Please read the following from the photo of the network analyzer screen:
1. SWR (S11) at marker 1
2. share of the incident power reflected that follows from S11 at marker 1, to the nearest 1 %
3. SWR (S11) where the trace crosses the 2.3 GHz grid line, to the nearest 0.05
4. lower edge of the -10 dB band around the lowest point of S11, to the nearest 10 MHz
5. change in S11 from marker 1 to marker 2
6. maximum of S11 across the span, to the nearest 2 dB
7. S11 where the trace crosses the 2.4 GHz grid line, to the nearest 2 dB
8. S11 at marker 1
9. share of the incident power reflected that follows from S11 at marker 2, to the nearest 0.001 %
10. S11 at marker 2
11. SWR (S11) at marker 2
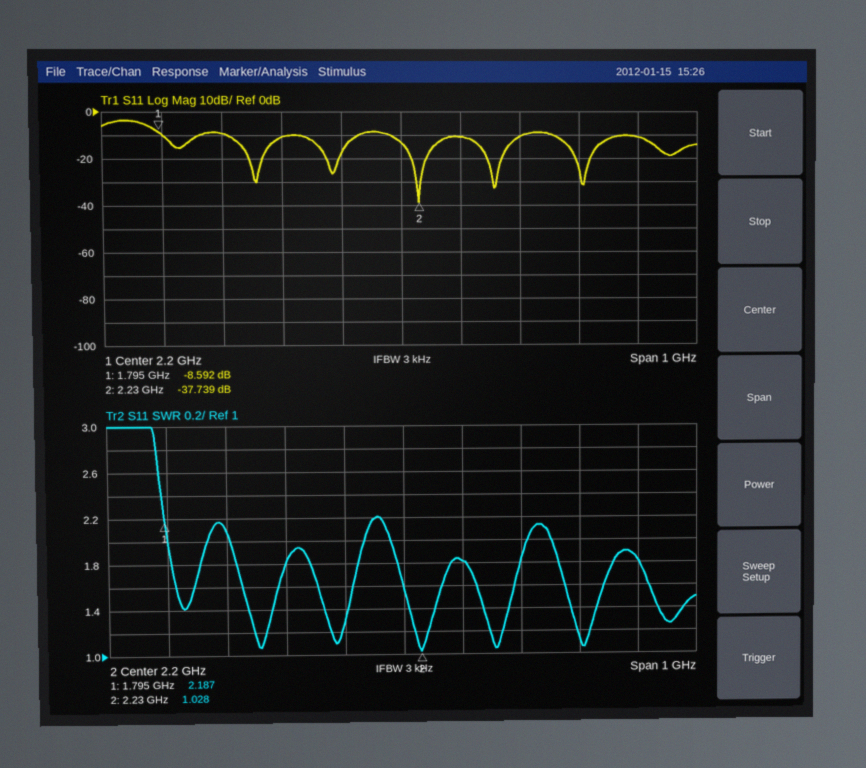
2.187
14 %
1.80
2.18 GHz
-29.147 dB
-4 dB
-10 dB
-8.592 dB
0.017 %
-37.739 dB
1.028
